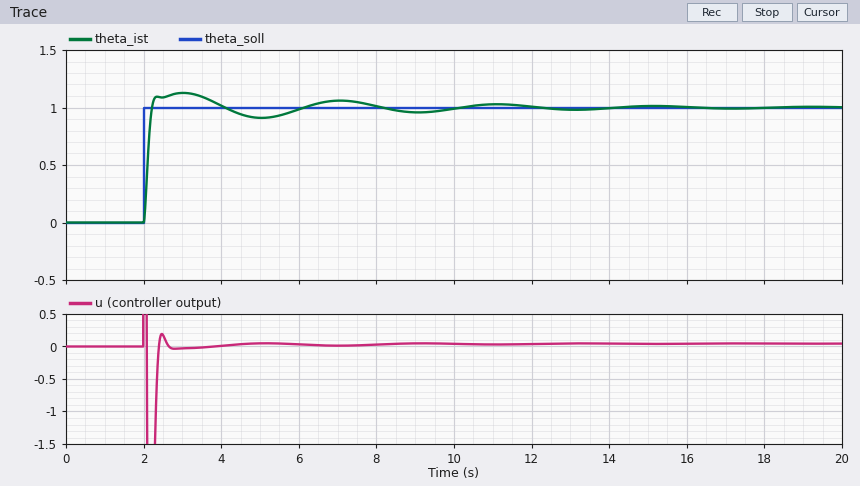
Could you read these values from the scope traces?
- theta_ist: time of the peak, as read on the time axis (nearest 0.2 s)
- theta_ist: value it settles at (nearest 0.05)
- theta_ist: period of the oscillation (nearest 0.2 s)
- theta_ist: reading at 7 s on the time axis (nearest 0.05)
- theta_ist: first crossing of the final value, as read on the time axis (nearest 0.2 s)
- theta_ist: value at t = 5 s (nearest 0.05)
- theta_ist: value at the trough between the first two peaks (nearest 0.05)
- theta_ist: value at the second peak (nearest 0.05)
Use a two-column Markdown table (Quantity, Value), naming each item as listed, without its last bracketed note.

| Quantity | Value |
|---|---|
| theta_ist: time of the peak, as read on the time axis | 3.0 s |
| theta_ist: value it settles at | 1.00 |
| theta_ist: period of the oscillation | 4.0 s |
| theta_ist: reading at 7 s on the time axis | 1.05 |
| theta_ist: first crossing of the final value, as read on the time axis | 2.2 s |
| theta_ist: value at t = 5 s | 0.90 |
| theta_ist: value at the trough between the first two peaks | 0.90 |
| theta_ist: value at the second peak | 1.05 |
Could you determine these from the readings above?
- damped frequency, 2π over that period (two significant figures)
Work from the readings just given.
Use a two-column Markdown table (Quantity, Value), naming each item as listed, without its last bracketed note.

| Quantity | Value |
|---|---|
| damped frequency, 2π over that period | 1.6 rad/s |
